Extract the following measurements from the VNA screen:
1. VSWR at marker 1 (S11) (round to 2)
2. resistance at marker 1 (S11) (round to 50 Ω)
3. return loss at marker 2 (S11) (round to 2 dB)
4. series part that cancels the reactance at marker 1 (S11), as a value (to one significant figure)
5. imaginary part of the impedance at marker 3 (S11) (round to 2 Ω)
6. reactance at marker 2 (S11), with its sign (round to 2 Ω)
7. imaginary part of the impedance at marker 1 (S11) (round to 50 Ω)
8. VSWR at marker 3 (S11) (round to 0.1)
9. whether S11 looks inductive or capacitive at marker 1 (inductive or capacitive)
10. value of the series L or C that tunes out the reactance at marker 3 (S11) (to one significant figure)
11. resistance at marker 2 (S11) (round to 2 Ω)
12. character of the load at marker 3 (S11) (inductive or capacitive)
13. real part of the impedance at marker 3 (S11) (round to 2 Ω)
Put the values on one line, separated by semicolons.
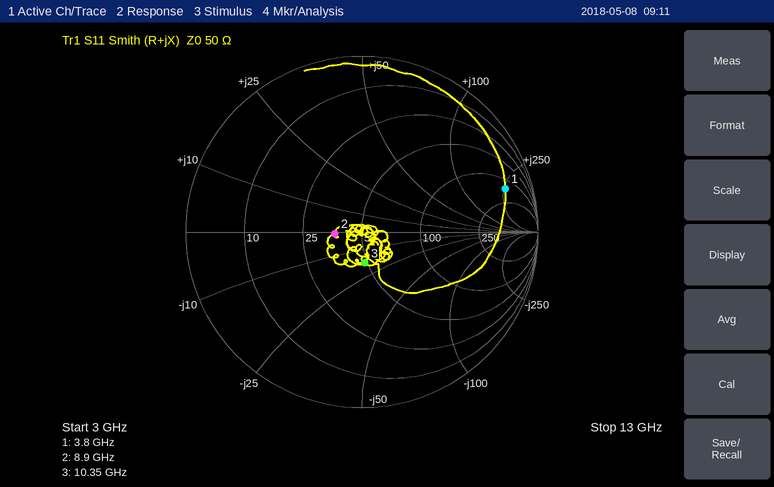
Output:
12; 150 Ω; 16 dB; 200 fF; -18 Ω; 0 Ω; +250 Ω; 1.4; inductive; 300 pH; 36 Ω; capacitive; 48 Ω
